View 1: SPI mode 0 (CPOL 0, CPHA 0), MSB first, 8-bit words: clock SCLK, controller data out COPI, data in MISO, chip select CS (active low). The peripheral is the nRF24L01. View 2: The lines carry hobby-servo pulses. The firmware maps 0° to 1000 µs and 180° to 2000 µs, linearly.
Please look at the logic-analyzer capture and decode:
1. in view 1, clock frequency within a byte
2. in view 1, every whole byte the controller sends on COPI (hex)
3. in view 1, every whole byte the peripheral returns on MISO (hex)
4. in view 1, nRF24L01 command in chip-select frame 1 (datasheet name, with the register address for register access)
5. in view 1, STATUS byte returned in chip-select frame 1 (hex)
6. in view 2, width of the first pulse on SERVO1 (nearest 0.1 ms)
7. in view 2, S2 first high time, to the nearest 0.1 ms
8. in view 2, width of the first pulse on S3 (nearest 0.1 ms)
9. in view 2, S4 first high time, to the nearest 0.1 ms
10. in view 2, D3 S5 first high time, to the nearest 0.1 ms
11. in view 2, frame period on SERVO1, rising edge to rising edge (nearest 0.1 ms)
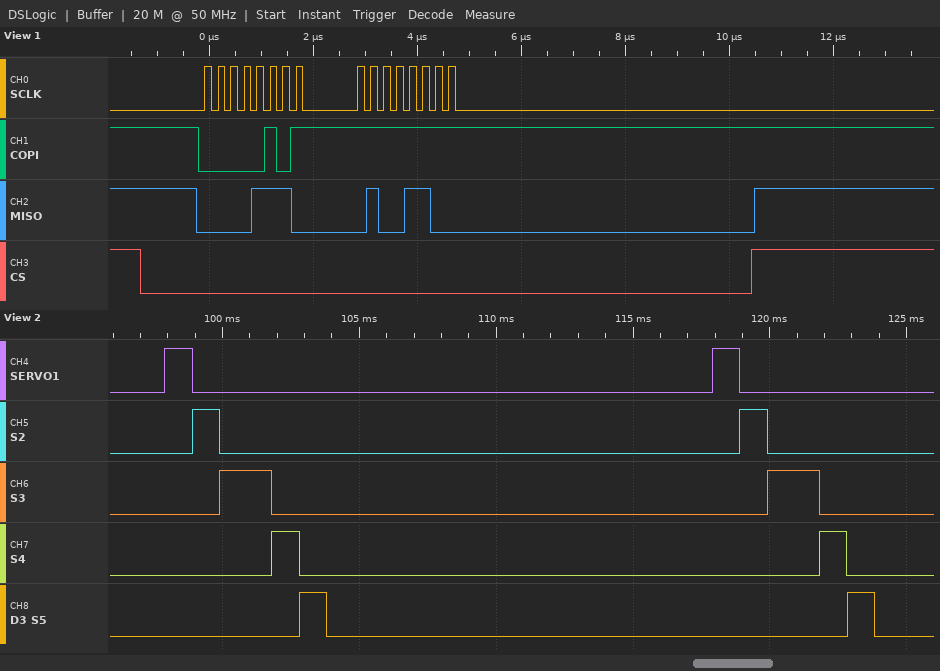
4 MHz
0x05 0xFF
0x0E 0x4C
R_REGISTER 0x05
0x0E
1.0 ms
1.0 ms
1.9 ms
1.0 ms
1.0 ms
20.0 ms
